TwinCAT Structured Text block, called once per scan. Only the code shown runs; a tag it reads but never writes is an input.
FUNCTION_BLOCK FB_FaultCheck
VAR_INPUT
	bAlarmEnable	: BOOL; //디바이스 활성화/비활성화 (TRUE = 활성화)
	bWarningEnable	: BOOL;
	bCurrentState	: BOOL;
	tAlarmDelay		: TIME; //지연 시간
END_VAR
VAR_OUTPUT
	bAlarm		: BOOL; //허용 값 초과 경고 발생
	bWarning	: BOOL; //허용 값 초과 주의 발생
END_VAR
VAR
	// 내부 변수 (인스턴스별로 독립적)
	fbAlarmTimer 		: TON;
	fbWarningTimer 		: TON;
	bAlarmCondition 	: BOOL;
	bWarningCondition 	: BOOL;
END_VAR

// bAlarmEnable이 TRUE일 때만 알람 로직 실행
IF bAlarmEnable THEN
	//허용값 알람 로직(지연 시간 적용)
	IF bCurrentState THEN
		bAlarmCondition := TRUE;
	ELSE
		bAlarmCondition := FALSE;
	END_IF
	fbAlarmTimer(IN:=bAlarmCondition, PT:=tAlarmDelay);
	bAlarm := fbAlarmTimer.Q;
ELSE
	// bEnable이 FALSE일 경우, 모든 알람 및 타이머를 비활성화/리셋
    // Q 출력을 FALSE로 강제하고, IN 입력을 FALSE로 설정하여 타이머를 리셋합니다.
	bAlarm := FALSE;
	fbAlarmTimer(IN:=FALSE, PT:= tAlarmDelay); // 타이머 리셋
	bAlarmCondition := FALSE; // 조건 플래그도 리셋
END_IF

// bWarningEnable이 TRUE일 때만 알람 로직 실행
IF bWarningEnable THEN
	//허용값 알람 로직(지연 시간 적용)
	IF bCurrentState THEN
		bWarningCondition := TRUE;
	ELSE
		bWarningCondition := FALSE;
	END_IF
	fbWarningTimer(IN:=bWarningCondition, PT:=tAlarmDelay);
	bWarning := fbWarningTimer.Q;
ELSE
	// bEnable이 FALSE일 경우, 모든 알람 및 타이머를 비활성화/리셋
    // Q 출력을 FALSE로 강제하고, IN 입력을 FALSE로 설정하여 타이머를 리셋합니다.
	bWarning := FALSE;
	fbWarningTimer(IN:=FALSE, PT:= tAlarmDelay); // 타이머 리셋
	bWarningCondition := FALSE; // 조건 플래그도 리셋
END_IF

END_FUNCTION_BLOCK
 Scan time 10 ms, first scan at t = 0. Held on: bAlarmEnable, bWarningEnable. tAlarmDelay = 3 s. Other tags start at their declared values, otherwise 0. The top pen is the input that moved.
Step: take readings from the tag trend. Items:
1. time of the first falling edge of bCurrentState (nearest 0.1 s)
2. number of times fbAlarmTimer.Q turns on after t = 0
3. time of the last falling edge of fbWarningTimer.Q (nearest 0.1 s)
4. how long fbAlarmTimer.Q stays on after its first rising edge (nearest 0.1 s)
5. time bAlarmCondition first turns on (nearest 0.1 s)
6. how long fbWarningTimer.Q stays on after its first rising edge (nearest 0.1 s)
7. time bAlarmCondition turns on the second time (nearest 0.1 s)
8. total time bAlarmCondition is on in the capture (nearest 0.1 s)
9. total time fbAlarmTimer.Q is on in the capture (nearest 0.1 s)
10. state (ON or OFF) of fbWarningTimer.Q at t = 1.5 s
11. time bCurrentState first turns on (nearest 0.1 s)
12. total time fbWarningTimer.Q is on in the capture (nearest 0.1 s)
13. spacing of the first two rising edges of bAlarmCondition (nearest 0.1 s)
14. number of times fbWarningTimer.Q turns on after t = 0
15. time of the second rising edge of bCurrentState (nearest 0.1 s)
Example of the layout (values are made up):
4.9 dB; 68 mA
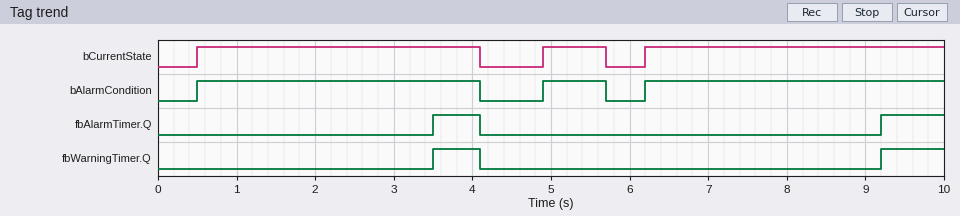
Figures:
4.1 s; 2; 4.1 s; 0.6 s; 0.5 s; 0.6 s; 4.9 s; 8.2 s; 1.4 s; OFF; 0.5 s; 1.4 s; 4.4 s; 2; 4.9 s
